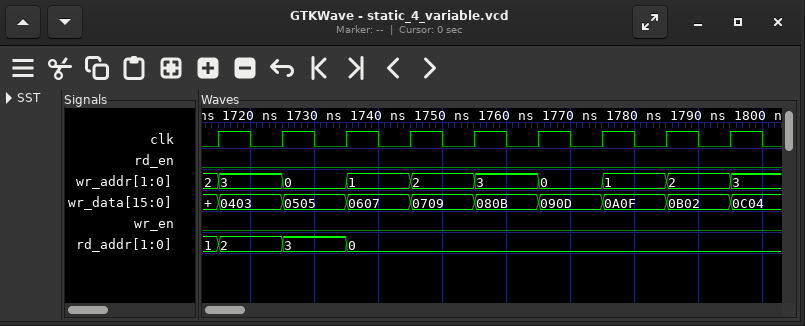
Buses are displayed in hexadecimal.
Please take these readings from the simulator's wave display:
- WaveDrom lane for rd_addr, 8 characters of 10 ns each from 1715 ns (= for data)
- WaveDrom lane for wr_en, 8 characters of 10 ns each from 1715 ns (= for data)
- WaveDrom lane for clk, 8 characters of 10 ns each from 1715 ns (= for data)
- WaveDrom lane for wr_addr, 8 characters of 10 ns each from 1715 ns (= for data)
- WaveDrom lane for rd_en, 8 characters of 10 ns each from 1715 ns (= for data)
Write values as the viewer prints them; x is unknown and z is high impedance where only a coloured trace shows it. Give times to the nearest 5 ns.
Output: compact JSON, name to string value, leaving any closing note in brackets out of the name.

{"WaveDrom lane for rd_addr, 8 characters of 10 ns each from 1715 ns": "{name: 'rd_addr', wave: '===.....', data: '2 3 0'}", "WaveDrom lane for wr_en, 8 characters of 10 ns each from 1715 ns": "{name: 'wr_en', wave: '0.......'}", "WaveDrom lane for clk, 8 characters of 10 ns each from 1715 ns": "{name: 'clk', wave: 'p.......'}", "WaveDrom lane for wr_addr, 8 characters of 10 ns each from 1715 ns": "{name: 'wr_addr', wave: '========', data: '3 0 1 2 3 0 1 2'}", "WaveDrom lane for rd_en, 8 characters of 10 ns each from 1715 ns": "{name: 'rd_en', wave: '0.......'}"}
